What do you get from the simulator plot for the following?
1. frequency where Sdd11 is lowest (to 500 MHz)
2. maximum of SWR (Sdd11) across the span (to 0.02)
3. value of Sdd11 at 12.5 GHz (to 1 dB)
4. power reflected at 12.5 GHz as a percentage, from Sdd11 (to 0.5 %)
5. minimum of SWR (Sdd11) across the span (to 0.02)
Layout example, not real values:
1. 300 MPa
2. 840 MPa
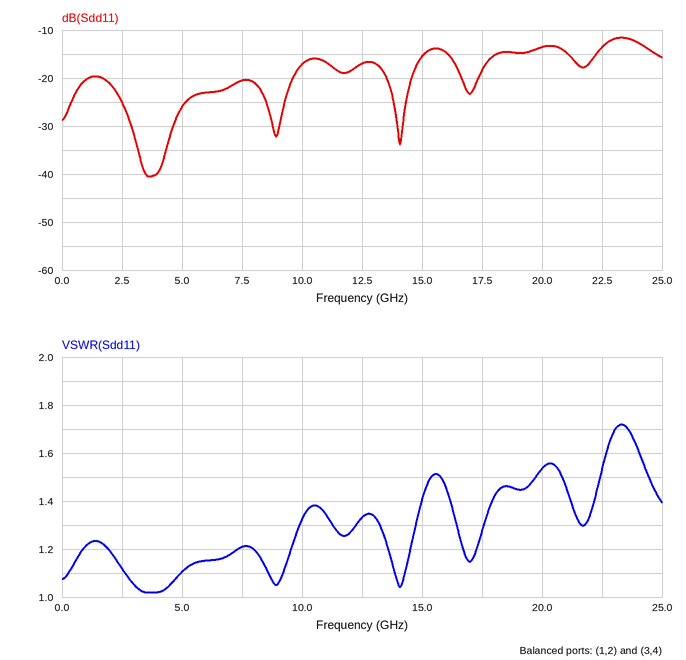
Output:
1. 3.5 GHz
2. 1.72
3. -17 dB
4. 2.0 %
5. 1.02
